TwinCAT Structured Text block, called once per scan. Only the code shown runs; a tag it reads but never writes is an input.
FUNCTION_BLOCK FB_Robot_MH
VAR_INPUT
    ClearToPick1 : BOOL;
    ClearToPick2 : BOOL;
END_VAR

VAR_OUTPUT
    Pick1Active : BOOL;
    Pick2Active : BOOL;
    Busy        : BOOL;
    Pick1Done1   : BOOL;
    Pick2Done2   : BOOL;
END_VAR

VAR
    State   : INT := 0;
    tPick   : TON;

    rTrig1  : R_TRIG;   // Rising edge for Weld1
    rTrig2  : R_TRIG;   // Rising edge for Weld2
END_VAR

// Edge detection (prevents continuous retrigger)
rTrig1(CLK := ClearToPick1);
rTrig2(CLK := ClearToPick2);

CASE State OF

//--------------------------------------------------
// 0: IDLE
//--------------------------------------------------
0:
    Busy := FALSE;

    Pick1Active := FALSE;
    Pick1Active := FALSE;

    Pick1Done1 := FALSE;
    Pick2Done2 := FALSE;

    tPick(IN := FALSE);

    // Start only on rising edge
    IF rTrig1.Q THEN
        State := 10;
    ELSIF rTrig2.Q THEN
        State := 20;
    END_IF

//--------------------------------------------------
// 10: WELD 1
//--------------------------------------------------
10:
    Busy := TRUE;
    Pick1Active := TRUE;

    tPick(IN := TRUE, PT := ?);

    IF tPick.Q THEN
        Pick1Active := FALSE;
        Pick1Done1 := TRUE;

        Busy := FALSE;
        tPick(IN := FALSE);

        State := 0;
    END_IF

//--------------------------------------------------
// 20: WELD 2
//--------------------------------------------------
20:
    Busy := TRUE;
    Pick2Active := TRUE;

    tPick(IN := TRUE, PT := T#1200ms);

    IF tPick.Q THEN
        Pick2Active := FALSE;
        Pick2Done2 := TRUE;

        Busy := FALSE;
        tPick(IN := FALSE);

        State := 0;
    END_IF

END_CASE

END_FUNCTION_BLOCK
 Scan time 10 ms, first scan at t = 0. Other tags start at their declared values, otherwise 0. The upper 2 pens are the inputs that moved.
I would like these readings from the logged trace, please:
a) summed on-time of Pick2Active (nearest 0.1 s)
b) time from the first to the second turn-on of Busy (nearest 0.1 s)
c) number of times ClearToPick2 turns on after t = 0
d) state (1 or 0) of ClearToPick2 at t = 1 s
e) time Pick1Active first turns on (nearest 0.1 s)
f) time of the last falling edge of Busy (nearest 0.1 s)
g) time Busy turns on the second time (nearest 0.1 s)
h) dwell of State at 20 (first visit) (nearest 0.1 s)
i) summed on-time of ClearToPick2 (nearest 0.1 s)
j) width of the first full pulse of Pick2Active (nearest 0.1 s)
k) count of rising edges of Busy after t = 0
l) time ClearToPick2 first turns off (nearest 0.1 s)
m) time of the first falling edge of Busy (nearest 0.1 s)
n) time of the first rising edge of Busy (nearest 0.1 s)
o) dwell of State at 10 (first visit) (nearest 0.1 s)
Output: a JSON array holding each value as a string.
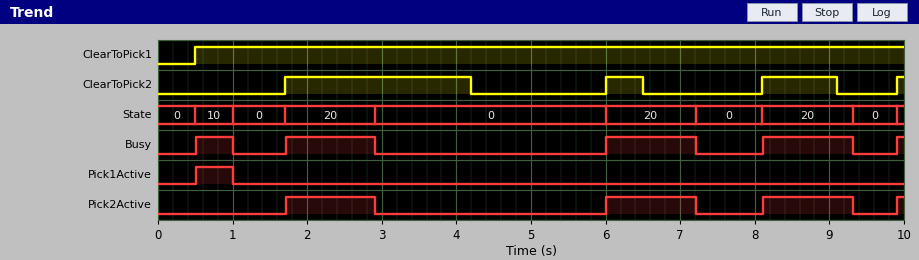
["3.7 s", "1.2 s", "4", "0", "0.5 s", "9.3 s", "1.7 s", "1.2 s", "4.1 s", "1.2 s", "5", "4.2 s", "1.0 s", "0.5 s", "0.5 s"]
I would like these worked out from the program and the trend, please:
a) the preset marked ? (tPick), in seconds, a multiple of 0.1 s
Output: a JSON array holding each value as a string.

["0.5 s"]
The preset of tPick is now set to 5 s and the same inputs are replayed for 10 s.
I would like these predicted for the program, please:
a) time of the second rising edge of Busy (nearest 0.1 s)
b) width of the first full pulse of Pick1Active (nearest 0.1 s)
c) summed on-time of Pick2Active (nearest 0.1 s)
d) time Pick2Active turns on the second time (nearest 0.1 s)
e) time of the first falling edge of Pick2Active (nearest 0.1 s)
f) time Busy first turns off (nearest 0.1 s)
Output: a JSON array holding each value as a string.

["6.0 s", "5.0 s", "2.5 s", "8.1 s", "7.2 s", "5.5 s"]
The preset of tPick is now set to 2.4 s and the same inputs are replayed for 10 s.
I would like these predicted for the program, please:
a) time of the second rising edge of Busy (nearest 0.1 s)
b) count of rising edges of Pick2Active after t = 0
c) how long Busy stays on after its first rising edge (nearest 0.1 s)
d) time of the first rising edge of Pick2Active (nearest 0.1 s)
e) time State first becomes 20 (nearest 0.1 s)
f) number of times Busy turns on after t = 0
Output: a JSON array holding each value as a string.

["6.0 s", "3", "2.4 s", "6.0 s", "6.0 s", "4"]
